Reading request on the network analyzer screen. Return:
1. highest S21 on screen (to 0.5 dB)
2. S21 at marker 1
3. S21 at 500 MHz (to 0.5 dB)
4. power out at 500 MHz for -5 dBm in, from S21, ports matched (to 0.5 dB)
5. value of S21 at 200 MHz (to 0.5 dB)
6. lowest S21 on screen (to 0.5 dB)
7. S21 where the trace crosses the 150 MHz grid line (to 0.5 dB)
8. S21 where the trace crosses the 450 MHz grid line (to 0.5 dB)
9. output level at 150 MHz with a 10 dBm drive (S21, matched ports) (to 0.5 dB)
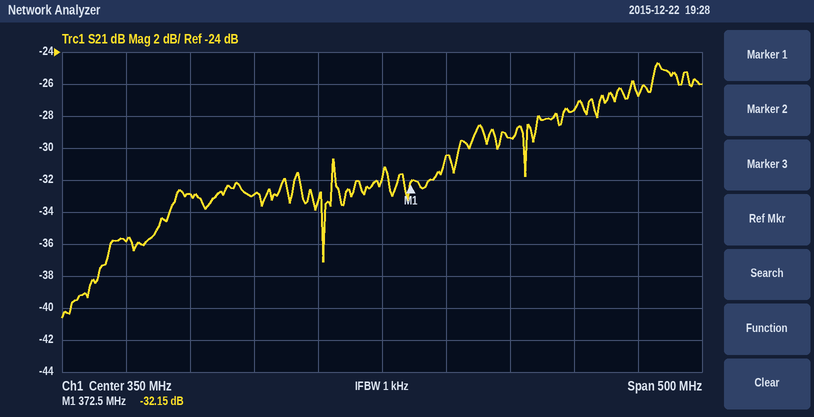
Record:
-24.5 dB
-32.15 dB
-27.5 dB
-32.5 dBm
-33.0 dB
-40.5 dB
-36.0 dB
-29.5 dB
-26.0 dBm
